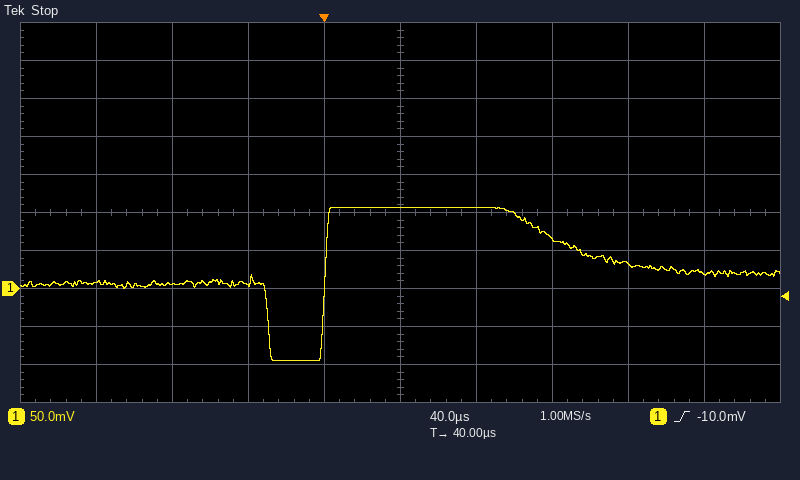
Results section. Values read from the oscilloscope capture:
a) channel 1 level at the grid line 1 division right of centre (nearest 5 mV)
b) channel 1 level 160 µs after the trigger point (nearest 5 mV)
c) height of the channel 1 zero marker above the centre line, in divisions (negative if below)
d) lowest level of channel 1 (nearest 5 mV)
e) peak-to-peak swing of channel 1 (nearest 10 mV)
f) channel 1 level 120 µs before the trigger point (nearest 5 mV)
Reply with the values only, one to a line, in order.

105 mV
30 mV
-2.0 div
-95 mV
200 mV
10 mV
